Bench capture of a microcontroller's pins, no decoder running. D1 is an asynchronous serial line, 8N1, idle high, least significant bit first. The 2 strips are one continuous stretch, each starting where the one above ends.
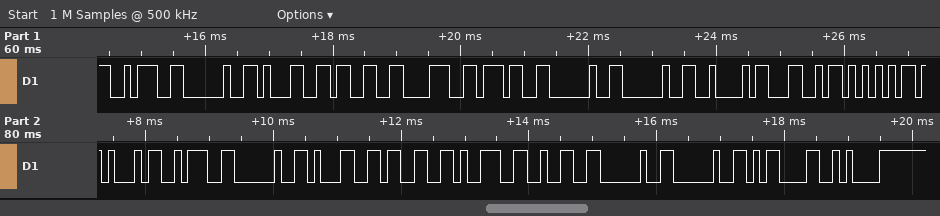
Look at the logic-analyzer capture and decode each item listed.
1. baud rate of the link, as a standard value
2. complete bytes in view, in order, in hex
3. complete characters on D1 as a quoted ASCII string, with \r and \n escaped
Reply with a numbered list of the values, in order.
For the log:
1. 9600 baud
2. 3A 20 31 33 38 37 20 20 42 4C 55 45 3A 20 31 33 39 32 20 20 0D 0A
3. ": 1387  BLUE: 1392  \r\n"
